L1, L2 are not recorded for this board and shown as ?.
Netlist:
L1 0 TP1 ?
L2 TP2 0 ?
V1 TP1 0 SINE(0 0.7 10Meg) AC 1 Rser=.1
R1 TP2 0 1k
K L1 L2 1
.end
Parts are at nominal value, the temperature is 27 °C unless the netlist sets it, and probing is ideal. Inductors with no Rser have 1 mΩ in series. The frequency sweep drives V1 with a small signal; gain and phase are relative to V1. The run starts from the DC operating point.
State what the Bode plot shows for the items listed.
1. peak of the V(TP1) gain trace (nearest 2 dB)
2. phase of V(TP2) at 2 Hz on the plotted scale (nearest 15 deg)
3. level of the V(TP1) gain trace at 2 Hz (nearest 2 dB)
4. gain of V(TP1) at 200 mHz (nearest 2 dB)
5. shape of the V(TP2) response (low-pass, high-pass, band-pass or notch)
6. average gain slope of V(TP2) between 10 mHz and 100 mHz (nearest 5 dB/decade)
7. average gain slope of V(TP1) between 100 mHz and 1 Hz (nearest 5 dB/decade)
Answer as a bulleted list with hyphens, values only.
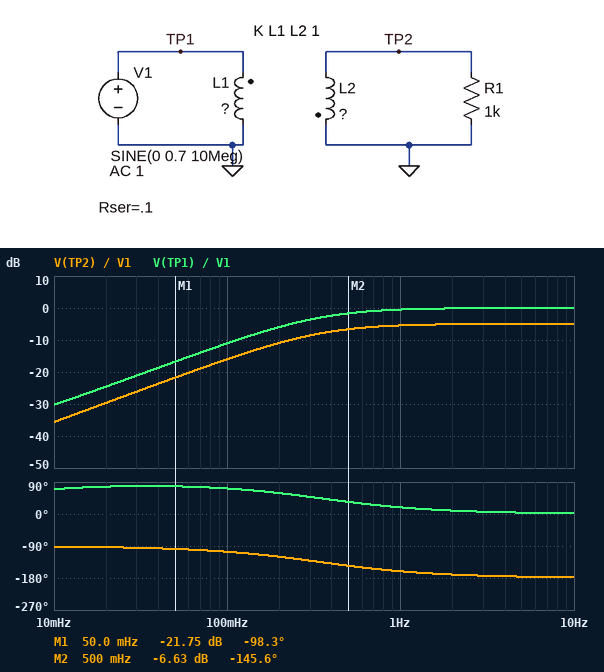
- 0 dB
- -165 deg
- 0 dB
- -6 dB
- high-pass
- 20 dB/decade
- 10 dB/decade
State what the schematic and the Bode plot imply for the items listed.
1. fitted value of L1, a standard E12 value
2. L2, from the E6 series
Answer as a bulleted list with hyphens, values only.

- 47 mH
- 15 mH
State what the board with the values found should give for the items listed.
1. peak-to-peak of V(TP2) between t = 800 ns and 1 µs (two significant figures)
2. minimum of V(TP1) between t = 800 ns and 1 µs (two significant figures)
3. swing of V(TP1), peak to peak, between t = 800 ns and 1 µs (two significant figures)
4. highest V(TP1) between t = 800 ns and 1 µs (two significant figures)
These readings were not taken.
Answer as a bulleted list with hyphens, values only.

- 790 mV
- -700 mV
- 1.4 V
- 700 mV
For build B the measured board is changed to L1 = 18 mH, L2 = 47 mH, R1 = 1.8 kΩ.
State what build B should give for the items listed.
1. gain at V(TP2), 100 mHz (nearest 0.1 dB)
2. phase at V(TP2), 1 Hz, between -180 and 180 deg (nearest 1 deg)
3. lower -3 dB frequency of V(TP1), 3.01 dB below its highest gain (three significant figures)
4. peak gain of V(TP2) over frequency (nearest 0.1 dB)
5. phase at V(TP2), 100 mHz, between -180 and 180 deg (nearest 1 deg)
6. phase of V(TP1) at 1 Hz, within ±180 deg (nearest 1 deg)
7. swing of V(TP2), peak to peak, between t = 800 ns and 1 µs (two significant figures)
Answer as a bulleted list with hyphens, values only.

- -14.9 dB
- -138 deg
- 893 mHz
- 4.2 dB
- -96 deg
- 41 deg
- 2.3 V
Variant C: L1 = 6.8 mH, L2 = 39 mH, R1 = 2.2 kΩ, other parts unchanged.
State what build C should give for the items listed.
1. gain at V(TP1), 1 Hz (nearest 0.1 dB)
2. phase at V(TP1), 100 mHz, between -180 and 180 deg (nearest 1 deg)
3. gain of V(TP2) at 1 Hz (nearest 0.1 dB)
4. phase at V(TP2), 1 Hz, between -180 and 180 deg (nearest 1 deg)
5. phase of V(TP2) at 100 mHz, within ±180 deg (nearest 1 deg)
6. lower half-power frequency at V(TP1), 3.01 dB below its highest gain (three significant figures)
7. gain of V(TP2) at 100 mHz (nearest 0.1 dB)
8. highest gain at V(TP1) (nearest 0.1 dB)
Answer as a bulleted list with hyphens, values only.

- -8.2 dB
- 74 deg
- -0.6 dB
- -113 deg
- -92 deg
- 2.36 Hz
- -19.9 dB
- 0 dB
